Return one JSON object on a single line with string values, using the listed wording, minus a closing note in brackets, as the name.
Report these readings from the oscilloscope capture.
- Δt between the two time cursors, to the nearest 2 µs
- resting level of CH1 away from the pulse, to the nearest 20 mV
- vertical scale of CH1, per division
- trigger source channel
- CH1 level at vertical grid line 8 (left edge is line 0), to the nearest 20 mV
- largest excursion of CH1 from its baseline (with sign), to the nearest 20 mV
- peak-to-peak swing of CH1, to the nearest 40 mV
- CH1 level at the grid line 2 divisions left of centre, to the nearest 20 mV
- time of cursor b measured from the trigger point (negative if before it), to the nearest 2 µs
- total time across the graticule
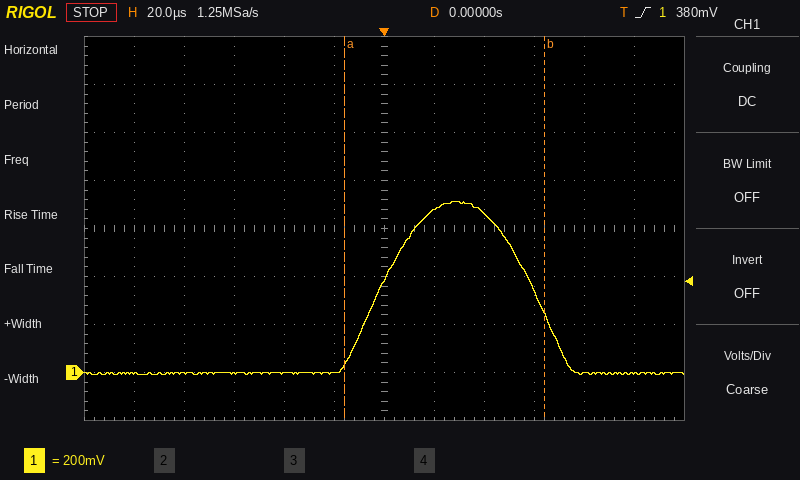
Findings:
{"Δt between the two time cursors, to the nearest 2 µs": "80 µs", "resting level of CH1 away from the pulse, to the nearest 20 mV": "0 mV", "vertical scale of CH1, per division": "200 mV", "trigger source channel": "CH1", "CH1 level at vertical grid line 8 (left edge is line 0), to the nearest 20 mV": "660 mV", "largest excursion of CH1 from its baseline (with sign), to the nearest 20 mV": "+720 mV", "peak-to-peak swing of CH1, to the nearest 40 mV": "720 mV", "CH1 level at the grid line 2 divisions left of centre, to the nearest 20 mV": "0 mV", "time of cursor b measured from the trigger point (negative if before it), to the nearest 2 µs": "+64 µs", "total time across the graticule": "240 µs"}
